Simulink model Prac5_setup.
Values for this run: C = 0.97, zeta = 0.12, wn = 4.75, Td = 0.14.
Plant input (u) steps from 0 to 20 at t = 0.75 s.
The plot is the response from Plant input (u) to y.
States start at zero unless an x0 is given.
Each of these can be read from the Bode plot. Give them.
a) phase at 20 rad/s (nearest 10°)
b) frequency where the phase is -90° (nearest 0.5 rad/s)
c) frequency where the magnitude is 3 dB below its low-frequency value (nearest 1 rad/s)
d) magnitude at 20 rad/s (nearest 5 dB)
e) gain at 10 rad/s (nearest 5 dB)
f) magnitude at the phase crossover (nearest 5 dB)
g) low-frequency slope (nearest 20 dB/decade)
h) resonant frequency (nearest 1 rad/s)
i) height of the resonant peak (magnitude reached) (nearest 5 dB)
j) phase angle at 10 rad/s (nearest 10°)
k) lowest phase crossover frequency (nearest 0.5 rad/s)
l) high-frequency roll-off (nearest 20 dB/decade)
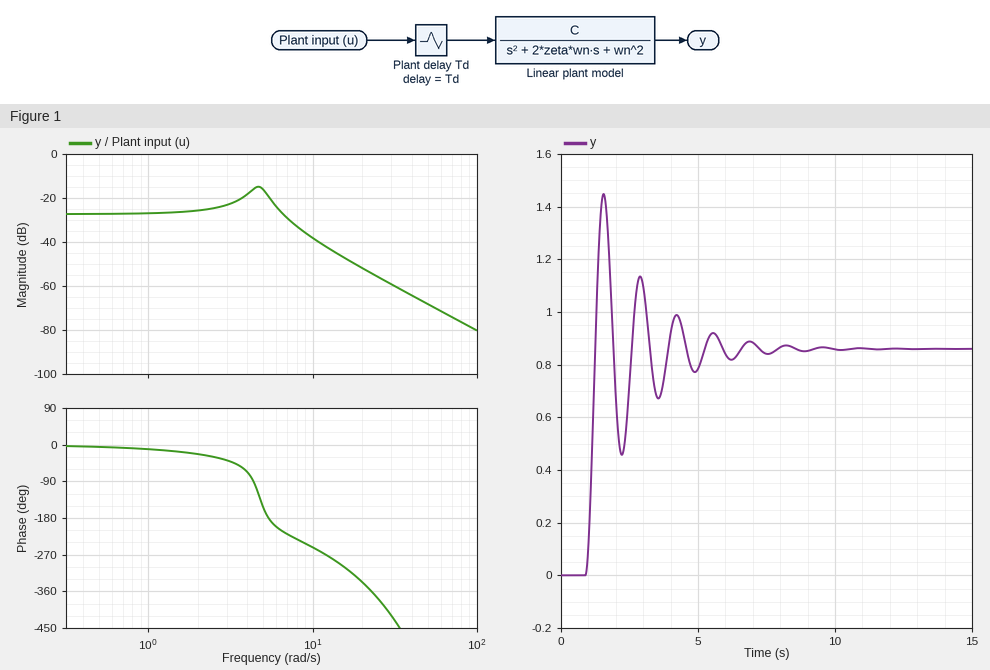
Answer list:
-340°
4.5 rad/s
7 rad/s
-50 dB
-40 dB
-20 dB
0 dB/decade
5 rad/s
-15 dB
-250°
5.5 rad/s
-40 dB/decade
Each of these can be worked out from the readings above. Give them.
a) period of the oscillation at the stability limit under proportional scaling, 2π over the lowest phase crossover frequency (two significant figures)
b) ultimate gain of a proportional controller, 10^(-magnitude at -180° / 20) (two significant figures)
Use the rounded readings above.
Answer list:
1.1 s
10
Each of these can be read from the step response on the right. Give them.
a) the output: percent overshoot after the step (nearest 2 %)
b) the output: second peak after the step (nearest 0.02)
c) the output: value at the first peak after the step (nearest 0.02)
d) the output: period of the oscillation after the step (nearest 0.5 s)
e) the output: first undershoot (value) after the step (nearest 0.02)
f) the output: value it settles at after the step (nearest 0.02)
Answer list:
68 %
1.14
1.44
1.5 s
0.46
0.86
